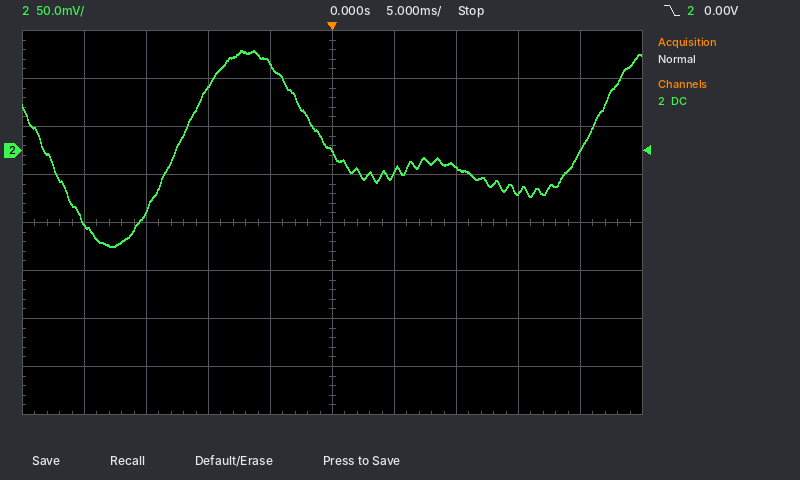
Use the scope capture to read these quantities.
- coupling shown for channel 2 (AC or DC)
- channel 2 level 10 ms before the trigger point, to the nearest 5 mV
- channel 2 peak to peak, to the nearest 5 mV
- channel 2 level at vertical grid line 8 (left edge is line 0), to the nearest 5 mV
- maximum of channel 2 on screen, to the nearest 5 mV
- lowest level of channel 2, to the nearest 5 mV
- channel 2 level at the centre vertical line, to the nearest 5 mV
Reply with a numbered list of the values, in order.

1. DC
2. 65 mV
3. 205 mV
4. -45 mV
5. 105 mV
6. -100 mV
7. 0 mV
